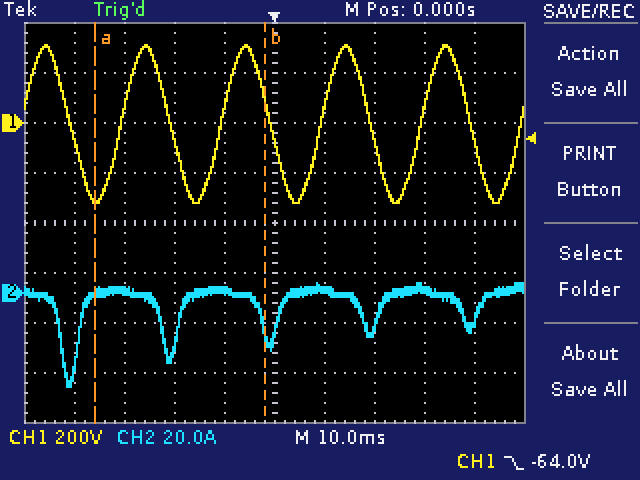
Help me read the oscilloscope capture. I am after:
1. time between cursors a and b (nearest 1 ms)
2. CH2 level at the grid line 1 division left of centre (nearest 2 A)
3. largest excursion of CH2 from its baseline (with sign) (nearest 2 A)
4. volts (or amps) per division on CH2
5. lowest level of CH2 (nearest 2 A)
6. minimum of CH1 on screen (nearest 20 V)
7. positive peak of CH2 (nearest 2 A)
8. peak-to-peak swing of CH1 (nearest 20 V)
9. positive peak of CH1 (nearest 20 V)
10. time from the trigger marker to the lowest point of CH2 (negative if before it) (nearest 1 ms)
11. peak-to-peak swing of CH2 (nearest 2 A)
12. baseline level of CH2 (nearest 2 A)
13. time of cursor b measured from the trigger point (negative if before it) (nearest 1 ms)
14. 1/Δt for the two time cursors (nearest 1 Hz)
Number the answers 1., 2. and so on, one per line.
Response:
1. 34 ms
2. 0 A
3. -38 A
4. 20 A
5. -38 A
6. -320 V
7. 4 A
8. 640 V
9. 320 V
10. -41 ms
11. 42 A
12. 0 A
13. -2 ms
14. 29 Hz
